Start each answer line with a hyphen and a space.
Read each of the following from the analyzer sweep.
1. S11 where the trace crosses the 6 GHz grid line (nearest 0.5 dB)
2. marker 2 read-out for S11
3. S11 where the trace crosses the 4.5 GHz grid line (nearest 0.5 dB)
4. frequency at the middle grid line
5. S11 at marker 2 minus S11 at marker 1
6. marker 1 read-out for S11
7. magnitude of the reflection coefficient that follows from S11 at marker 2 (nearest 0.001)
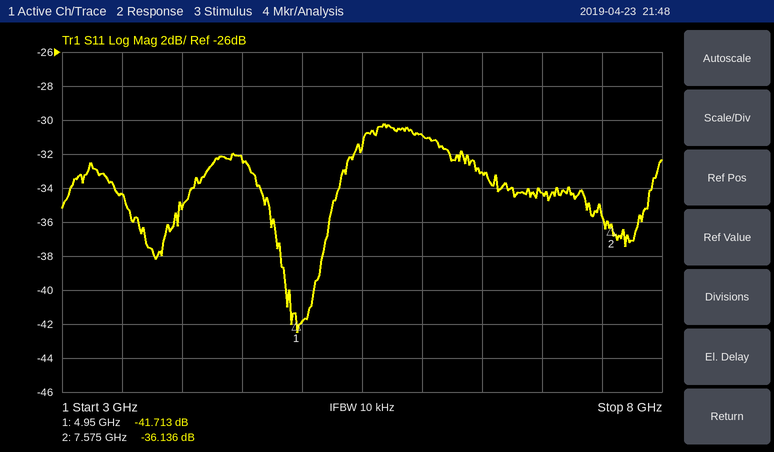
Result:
- -31.0 dB
- -36.136 dB
- -32.5 dB
- 5.5 GHz
- 5.577 dB
- -41.713 dB
- 0.016
